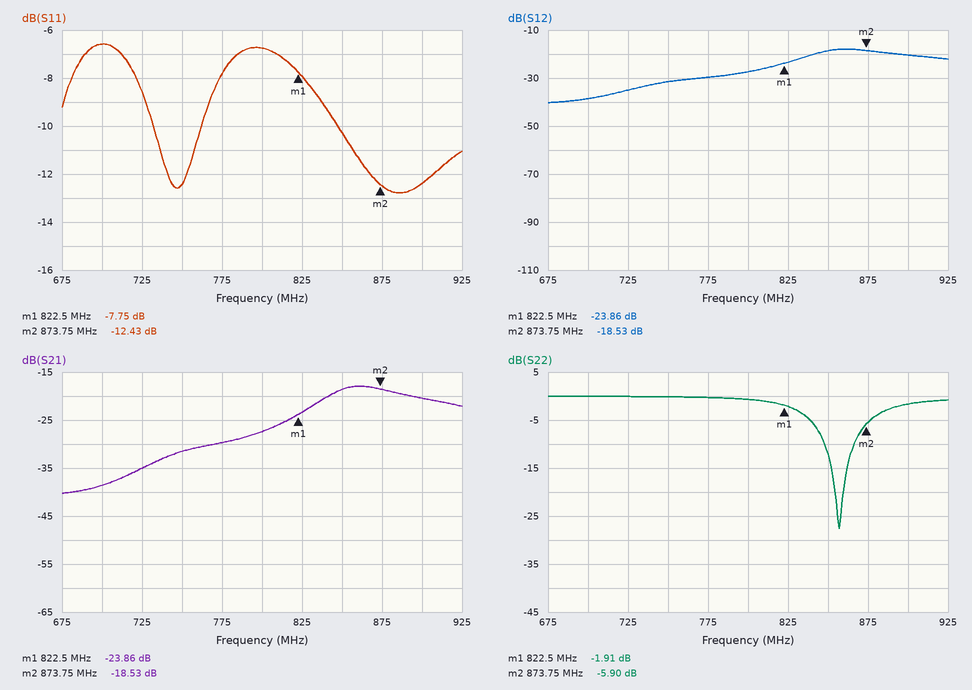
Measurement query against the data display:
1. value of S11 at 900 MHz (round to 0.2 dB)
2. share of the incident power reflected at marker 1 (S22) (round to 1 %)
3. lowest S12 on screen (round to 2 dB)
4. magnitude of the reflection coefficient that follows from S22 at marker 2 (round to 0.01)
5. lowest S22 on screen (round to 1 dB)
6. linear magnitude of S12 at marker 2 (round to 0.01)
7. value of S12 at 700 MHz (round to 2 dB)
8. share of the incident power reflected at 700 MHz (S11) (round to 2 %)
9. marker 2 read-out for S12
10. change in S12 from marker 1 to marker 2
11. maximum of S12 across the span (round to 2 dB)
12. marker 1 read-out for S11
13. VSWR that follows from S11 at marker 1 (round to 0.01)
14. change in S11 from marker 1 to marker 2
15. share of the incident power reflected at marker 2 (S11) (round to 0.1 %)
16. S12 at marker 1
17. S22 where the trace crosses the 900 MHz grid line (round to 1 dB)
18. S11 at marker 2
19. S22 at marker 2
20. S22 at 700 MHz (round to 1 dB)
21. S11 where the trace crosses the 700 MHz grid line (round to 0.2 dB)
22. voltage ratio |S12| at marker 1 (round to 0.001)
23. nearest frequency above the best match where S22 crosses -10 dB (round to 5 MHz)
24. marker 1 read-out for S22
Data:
-12.4 dB
64 %
-40 dB
0.51
-28 dB
0.12
-38 dB
22 %
-18.53 dB
5.33 dB
-18 dB
-7.75 dB
2.39
-4.68 dB
5.7 %
-23.86 dB
-2 dB
-12.43 dB
-5.90 dB
0 dB
-6.6 dB
0.064
865 MHz
-1.91 dB
